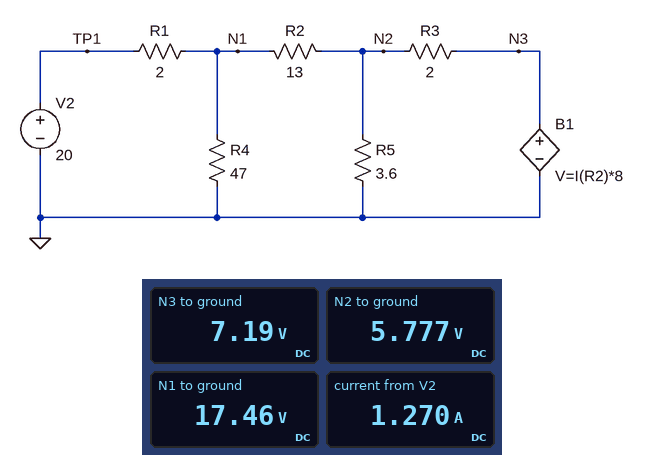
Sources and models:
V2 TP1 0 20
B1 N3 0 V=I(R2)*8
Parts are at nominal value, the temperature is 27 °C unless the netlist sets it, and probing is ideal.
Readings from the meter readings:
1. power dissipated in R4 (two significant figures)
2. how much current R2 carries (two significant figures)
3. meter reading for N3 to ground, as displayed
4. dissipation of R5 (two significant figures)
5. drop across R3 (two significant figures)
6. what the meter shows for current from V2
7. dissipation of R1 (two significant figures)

6.5 W
900 mA
7.19 V
9.3 W
1.4 V
1.270 A
3.2 W
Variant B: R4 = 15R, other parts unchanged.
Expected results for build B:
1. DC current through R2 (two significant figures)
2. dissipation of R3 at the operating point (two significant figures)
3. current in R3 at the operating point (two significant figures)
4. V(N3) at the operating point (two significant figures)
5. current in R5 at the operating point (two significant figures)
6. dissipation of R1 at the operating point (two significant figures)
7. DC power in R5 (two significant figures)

830 mA
860 mW
650 mA
6.7 V
1.5 A
7.3 W
8.0 W
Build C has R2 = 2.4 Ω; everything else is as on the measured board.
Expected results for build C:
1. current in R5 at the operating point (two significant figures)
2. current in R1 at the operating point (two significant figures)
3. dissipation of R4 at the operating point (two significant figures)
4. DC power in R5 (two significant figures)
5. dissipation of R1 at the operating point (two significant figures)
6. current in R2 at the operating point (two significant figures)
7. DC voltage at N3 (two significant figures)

3.2 A
2.1 A
5.3 W
37 W
9.0 W
1.8 A
14 V
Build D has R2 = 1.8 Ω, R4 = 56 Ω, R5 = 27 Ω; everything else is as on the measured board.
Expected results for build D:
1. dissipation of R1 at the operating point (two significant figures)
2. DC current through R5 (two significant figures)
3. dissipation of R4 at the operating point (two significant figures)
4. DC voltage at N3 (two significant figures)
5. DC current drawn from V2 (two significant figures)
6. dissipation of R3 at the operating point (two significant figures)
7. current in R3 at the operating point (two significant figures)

6.3 W
510 mA
4.8 W
12 V
1.8 A
1.9 W
970 mA
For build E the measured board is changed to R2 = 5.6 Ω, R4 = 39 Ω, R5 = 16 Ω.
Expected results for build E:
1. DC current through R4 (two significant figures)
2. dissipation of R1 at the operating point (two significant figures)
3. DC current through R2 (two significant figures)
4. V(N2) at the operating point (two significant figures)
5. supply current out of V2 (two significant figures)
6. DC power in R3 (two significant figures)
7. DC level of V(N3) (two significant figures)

430 mA
5.1 W
1.2 A
10 V
1.6 A
530 mW
9.3 V
